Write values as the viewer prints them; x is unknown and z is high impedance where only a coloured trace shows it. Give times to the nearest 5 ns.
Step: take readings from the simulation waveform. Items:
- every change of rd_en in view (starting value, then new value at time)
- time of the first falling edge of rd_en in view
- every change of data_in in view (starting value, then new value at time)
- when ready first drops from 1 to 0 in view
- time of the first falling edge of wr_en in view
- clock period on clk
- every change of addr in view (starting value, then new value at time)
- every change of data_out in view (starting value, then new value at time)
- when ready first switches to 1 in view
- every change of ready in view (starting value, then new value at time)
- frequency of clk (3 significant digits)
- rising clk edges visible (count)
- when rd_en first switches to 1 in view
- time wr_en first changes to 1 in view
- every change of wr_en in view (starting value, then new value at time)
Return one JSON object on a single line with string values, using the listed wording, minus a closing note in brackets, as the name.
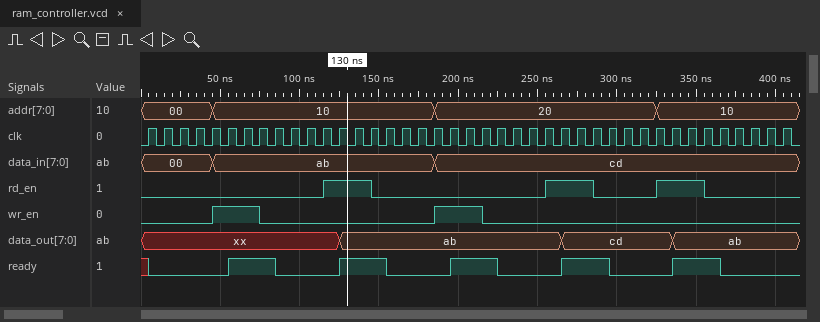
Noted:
{"every change of rd_en in view": "0, 1 at 115 ns, 0 at 145 ns, 1 at 255 ns, 0 at 285 ns, 1 at 325 ns, 0 at 355 ns", "time of the first falling edge of rd_en in view": "145 ns", "every change of data_in in view": "00, ab at 45 ns, cd at 185 ns", "when ready first drops from 1 to 0 in view": "85 ns", "time of the first falling edge of wr_en in view": "75 ns", "clock period on clk": "10 ns", "every change of addr in view": "00, 10 at 45 ns, 20 at 185 ns, 10 at 325 ns", "every change of data_out in view": "xx, ab at 125 ns, cd at 265 ns, ab at 335 ns", "when ready first switches to 1 in view": "55 ns", "every change of ready in view": "x, 0 at 5 ns, 1 at 55 ns, 0 at 85 ns, 1 at 125 ns, 0 at 155 ns, 1 at 195 ns, 0 at 225 ns, 1 at 265 ns, 0 at 295 ns, 1 at 335 ns, 0 at 365 ns", "frequency of clk": "100 MHz", "rising clk edges visible": "41", "when rd_en first switches to 1 in view": "115 ns", "time wr_en first changes to 1 in view": "45 ns", "every change of wr_en in view": "0, 1 at 45 ns, 0 at 75 ns, 1 at 185 ns, 0 at 215 ns"}
